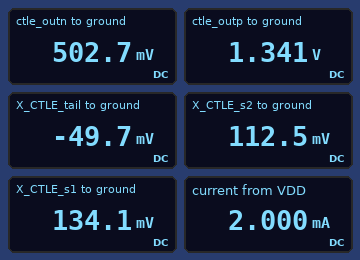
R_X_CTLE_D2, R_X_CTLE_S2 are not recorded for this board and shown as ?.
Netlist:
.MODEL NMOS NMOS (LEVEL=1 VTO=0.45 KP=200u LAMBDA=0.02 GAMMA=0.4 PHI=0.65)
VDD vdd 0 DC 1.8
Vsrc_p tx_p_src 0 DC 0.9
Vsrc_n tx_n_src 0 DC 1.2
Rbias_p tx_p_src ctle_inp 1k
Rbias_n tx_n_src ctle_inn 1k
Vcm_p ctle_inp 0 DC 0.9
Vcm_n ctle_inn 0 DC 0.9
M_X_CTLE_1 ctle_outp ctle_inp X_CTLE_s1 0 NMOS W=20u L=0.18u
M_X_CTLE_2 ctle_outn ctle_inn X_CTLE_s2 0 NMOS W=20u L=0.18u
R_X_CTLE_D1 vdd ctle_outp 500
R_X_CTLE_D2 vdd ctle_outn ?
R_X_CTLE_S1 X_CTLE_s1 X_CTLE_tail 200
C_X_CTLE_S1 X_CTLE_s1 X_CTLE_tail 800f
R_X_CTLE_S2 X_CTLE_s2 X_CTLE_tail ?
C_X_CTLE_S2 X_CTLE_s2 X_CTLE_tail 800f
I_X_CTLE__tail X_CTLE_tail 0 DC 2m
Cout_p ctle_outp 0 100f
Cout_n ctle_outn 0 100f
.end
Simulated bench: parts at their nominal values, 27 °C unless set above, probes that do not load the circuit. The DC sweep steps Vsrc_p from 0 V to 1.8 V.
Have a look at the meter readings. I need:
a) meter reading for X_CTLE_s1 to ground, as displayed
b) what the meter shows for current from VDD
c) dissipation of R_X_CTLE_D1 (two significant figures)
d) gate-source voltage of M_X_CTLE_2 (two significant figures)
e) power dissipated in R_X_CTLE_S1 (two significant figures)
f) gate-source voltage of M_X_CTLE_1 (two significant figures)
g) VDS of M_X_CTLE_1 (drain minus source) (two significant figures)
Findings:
134.1 mV
2.000 mA
420 µW
790 mV
170 µW
770 mV
1.2 V
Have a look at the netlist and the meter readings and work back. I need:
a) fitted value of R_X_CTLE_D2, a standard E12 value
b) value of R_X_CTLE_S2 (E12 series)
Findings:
1.2 kΩ
150 Ω
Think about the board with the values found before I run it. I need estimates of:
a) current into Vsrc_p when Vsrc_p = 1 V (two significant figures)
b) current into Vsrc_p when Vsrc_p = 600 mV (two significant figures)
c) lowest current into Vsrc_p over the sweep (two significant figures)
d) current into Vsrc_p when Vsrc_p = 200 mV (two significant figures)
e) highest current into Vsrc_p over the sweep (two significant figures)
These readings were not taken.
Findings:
-100 µA
300 µA
-900 µA
700 µA
900 µA
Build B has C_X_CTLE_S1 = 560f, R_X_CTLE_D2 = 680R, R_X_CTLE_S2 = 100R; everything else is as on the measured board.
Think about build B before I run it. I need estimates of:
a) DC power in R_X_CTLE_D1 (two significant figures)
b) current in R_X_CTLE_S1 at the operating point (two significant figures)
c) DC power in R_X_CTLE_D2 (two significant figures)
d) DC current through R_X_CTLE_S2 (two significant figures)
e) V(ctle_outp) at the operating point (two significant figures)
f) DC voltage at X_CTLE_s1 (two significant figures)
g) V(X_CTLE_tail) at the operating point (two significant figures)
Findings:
330 µW
820 µA
950 µW
1.2 mA
1.4 V
150 mV
-16 mV
